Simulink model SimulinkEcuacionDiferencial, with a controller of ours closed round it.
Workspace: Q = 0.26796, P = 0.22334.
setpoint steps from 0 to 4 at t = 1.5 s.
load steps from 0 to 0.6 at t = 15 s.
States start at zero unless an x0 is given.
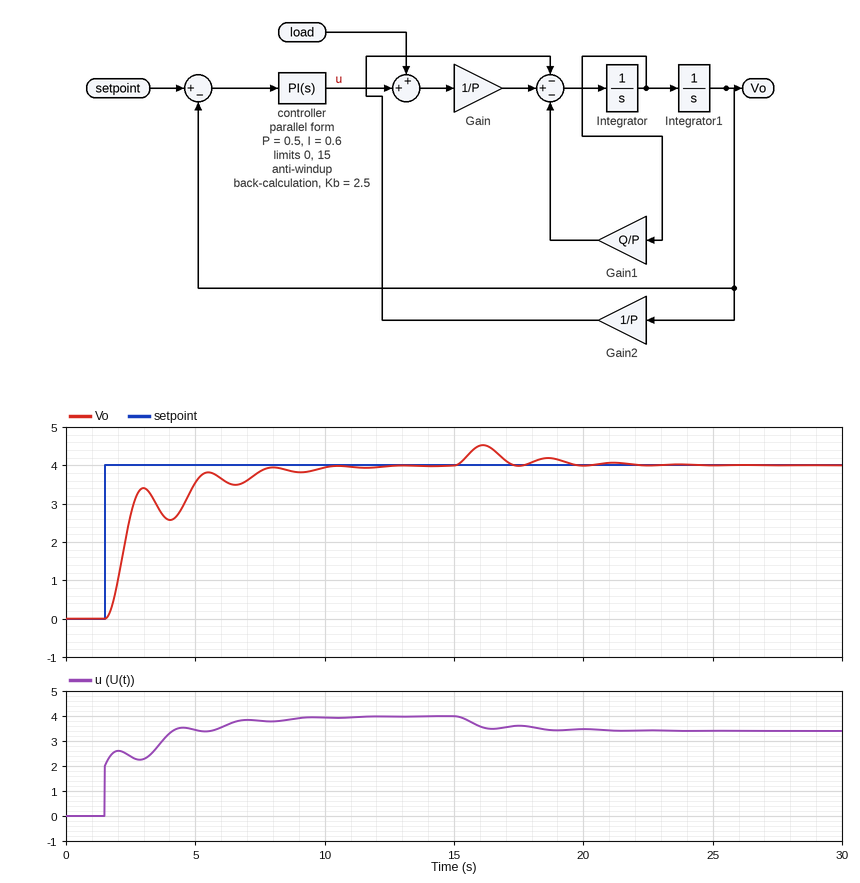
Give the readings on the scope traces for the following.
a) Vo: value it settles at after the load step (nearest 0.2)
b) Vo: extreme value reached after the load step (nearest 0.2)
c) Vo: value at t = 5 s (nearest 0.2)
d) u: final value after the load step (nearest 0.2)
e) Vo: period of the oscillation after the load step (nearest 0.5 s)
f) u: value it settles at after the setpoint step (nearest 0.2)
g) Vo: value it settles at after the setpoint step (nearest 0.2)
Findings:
4.0
4.6
3.6
3.4
2.5 s
4.0
4.0
